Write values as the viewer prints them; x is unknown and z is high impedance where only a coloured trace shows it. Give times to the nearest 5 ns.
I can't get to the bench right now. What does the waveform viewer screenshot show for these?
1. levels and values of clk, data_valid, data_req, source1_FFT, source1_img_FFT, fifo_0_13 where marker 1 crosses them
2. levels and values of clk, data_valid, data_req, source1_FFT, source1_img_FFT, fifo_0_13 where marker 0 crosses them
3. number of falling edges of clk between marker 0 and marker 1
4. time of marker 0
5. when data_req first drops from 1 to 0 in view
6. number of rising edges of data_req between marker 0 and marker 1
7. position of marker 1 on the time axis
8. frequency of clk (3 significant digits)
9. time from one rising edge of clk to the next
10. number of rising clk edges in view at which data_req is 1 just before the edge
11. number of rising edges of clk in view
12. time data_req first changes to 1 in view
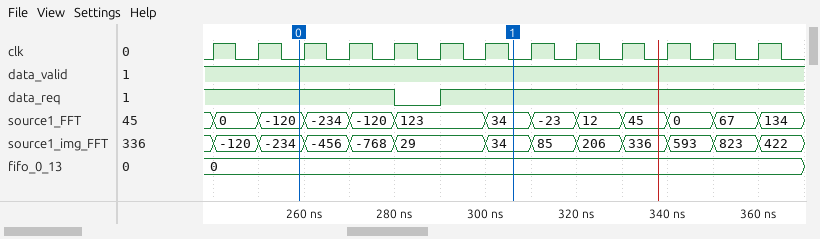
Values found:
clk=0, data_valid=1, data_req=1, source1_FFT=34, source1_img_FFT=34, fifo_0_13=0
clk=0, data_valid=1, data_req=1, source1_FFT=-120, source1_img_FFT=-234, fifo_0_13=0
5
260 ns
280 ns
1
305 ns
100 MHz
10 ns
12
13
290 ns
